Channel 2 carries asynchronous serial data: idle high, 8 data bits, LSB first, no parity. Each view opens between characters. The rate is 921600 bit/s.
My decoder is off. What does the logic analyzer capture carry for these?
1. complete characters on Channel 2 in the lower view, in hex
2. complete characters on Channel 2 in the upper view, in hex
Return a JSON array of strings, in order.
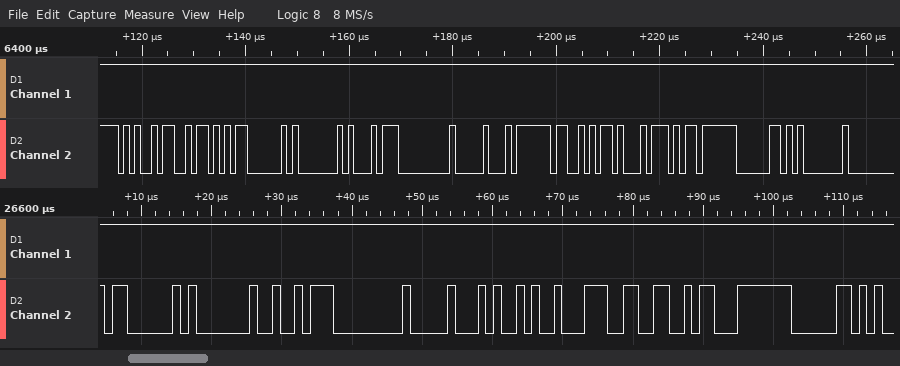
["03, 01, D2, 00, 10, 29, 9C, A6, FC, 60", "A5, 5A, 03, 01, D1, 00, 10, BF, 6A, 74, FB, 60, 01"]
